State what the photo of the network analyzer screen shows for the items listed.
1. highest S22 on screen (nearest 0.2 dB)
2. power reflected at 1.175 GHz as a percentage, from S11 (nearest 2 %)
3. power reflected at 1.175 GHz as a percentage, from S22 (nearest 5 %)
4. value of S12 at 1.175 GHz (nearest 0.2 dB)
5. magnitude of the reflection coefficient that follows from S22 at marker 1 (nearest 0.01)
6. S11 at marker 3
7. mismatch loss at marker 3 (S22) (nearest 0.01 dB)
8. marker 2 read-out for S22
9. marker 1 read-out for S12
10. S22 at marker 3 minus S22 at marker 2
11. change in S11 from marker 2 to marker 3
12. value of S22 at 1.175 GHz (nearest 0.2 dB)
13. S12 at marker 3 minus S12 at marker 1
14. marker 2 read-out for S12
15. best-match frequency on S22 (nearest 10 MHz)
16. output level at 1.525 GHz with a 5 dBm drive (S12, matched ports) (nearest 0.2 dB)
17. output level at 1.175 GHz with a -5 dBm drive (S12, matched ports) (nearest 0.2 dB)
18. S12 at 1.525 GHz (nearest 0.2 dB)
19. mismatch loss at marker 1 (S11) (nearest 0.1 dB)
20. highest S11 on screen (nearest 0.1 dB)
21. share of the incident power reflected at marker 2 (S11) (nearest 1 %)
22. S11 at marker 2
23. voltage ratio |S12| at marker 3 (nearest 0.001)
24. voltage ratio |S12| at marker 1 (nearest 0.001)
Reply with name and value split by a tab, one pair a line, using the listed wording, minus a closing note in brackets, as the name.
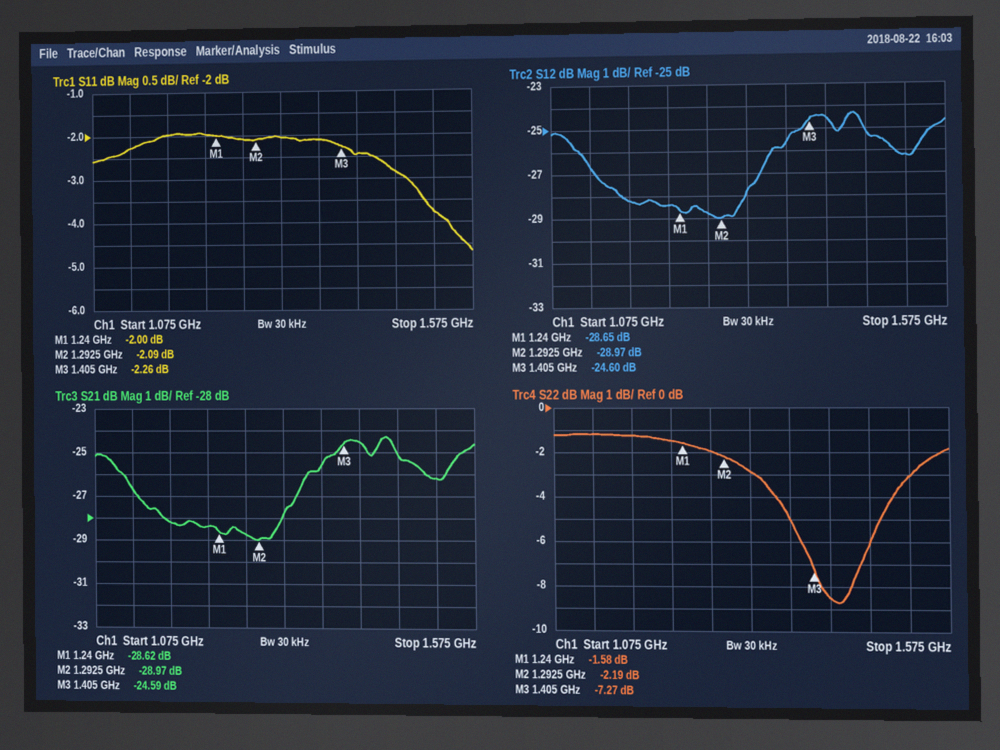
highest S22 on screen	-1.2 dB
power reflected at 1.175 GHz as a percentage, from S11	64 %
power reflected at 1.175 GHz as a percentage, from S22	75 %
value of S12 at 1.175 GHz	-28.2 dB
magnitude of the reflection coefficient that follows from S22 at marker 1	0.83
S11 at marker 3	-2.26 dB
mismatch loss at marker 3 (S22)	0.90 dB
marker 2 read-out for S22	-2.19 dB
marker 1 read-out for S12	-28.65 dB
S22 at marker 3 minus S22 at marker 2	-5.08 dB
change in S11 from marker 2 to marker 3	-0.17 dB
value of S22 at 1.175 GHz	-1.2 dB
S12 at marker 3 minus S12 at marker 1	4.05 dB
marker 2 read-out for S12	-28.97 dB
best-match frequency on S22	1.44 GHz
output level at 1.525 GHz with a 5 dBm drive (S12, matched ports)	-21.2 dBm
output level at 1.175 GHz with a -5 dBm drive (S12, matched ports)	-33.2 dBm
S12 at 1.525 GHz	-26.2 dB
mismatch loss at marker 1 (S11)	4.3 dB
highest S11 on screen	-1.9 dB
share of the incident power reflected at marker 2 (S11)	62 %
S11 at marker 2	-2.09 dB
voltage ratio |S12| at marker 3	0.059
voltage ratio |S12| at marker 1	0.037
